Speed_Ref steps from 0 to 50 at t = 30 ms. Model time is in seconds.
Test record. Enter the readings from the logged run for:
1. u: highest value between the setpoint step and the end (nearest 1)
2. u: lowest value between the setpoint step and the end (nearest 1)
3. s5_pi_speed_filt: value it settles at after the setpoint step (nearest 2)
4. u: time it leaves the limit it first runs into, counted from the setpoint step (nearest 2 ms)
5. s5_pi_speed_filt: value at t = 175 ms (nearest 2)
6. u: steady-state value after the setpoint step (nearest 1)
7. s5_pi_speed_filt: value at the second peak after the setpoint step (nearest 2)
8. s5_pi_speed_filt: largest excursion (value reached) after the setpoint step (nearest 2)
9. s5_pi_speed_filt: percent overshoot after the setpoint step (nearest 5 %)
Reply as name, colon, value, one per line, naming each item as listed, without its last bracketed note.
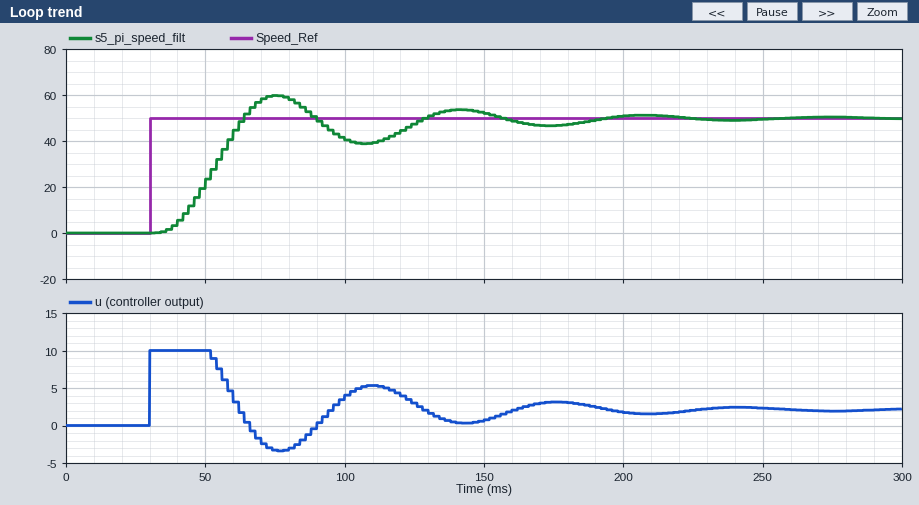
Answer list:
u: highest value between the setpoint step and the end: 10
u: lowest value between the setpoint step and the end: -3
s5_pi_speed_filt: value it settles at after the setpoint step: 50
u: time it leaves the limit it first runs into, counted from the setpoint step: 22 ms
s5_pi_speed_filt: value at t = 175 ms: 46
u: steady-state value after the setpoint step: 2
s5_pi_speed_filt: value at the second peak after the setpoint step: 54
s5_pi_speed_filt: largest excursion (value reached) after the setpoint step: 60
s5_pi_speed_filt: percent overshoot after the setpoint step: 20 %
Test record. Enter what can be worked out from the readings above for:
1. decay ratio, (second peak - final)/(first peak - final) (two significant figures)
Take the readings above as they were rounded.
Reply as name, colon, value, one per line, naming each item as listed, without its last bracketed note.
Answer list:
decay ratio, (second peak - final)/(first peak - final): 0.40
